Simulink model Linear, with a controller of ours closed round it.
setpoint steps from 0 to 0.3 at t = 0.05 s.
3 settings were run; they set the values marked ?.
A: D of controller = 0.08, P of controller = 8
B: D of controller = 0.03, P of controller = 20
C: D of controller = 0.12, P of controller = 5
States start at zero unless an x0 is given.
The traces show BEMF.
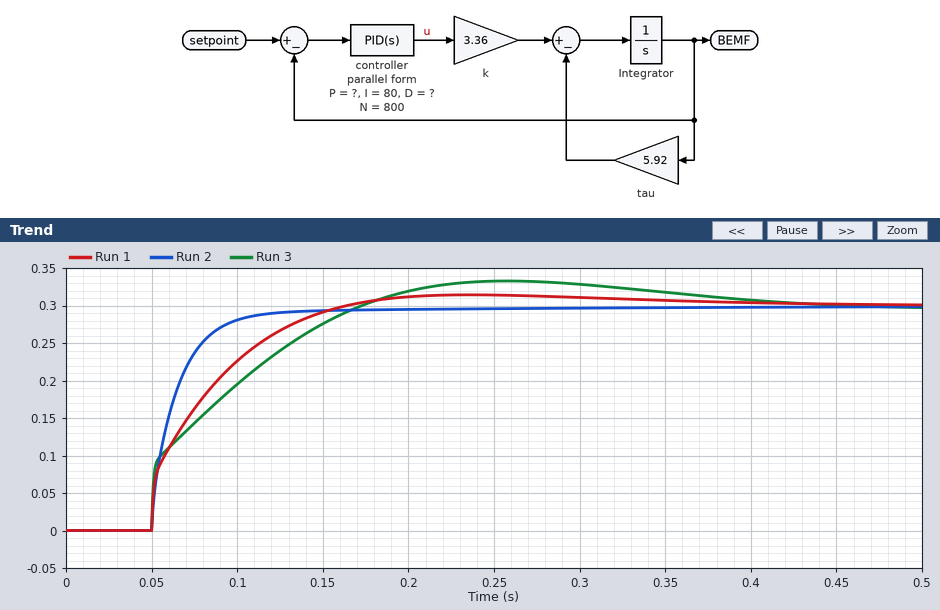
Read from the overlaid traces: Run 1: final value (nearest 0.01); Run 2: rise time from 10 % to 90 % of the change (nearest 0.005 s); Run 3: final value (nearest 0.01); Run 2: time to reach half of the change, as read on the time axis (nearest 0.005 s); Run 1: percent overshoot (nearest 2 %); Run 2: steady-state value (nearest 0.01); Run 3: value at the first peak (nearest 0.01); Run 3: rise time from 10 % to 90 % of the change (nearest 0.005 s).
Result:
0.30
0.040 s
0.30
0.060 s
4 %
0.30
0.33
0.095 s
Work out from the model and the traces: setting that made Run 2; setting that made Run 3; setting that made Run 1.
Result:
B
C
A
